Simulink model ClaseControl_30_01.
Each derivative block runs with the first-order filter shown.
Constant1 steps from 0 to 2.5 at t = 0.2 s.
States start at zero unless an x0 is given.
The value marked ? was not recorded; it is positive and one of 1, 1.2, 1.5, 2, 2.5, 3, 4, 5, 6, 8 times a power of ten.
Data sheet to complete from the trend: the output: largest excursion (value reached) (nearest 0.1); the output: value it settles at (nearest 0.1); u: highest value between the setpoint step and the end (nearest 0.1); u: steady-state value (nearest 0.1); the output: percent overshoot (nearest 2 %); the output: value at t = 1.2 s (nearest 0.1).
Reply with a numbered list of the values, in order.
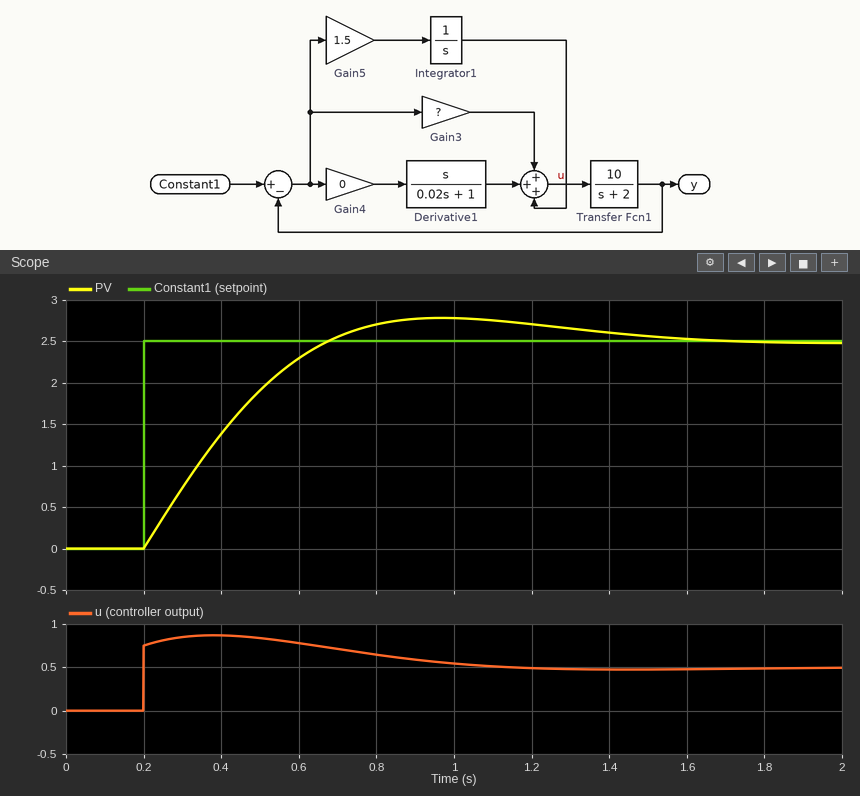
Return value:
1. 2.8
2. 2.5
3. 0.9
4. 0.5
5. 12 %
6. 2.7
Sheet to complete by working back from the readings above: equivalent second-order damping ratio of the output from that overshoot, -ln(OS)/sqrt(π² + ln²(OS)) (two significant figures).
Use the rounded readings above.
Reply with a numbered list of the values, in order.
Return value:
1. 0.56
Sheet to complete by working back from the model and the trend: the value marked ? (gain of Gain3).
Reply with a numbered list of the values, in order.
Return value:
1. 0.3
